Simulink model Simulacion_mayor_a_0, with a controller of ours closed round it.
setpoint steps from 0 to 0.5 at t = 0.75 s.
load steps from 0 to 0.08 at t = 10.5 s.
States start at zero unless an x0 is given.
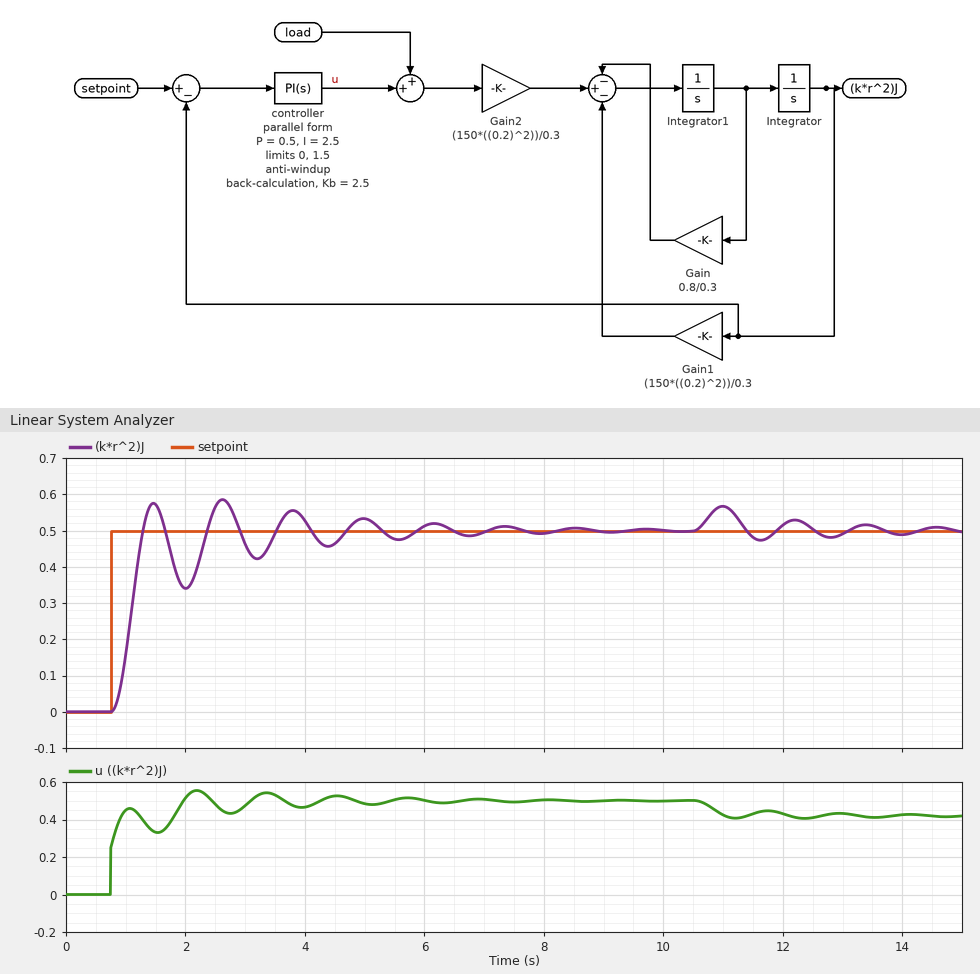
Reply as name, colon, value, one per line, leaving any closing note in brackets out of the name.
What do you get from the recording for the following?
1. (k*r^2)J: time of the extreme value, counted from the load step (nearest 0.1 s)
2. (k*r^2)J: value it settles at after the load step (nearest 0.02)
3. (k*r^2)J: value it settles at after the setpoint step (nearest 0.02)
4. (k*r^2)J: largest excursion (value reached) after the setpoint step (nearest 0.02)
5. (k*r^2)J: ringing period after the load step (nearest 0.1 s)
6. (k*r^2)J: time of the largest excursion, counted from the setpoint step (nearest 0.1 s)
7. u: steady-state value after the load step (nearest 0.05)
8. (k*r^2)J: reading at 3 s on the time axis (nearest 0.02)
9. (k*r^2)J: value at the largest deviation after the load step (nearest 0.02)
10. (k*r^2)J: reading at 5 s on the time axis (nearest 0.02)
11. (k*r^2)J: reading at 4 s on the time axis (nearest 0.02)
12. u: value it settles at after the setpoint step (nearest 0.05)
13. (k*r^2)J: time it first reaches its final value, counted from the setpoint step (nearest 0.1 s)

(k*r^2)J: time of the extreme value, counted from the load step: 0.5 s
(k*r^2)J: value it settles at after the load step: 0.50
(k*r^2)J: value it settles at after the setpoint step: 0.50
(k*r^2)J: largest excursion (value reached) after the setpoint step: 0.58
(k*r^2)J: ringing period after the load step: 1.2 s
(k*r^2)J: time of the largest excursion, counted from the setpoint step: 1.9 s
u: steady-state value after the load step: 0.40
(k*r^2)J: reading at 3 s on the time axis: 0.46
(k*r^2)J: value at the largest deviation after the load step: 0.56
(k*r^2)J: reading at 5 s on the time axis: 0.54
(k*r^2)J: reading at 4 s on the time axis: 0.52
u: value it settles at after the setpoint step: 0.50
(k*r^2)J: time it first reaches its final value, counted from the setpoint step: 0.5 s
